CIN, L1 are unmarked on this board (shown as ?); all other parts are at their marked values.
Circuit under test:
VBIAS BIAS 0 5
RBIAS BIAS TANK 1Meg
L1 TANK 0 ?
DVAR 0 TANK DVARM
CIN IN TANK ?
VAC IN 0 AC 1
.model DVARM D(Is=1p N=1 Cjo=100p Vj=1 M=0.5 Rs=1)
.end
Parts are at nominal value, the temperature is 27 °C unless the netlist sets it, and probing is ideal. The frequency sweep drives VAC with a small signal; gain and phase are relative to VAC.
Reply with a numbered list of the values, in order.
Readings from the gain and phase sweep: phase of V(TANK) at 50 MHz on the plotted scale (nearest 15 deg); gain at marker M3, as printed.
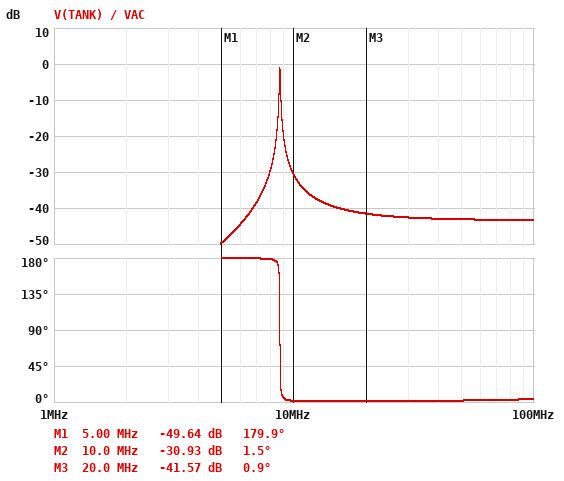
1. 0 deg
2. -41.57 dB
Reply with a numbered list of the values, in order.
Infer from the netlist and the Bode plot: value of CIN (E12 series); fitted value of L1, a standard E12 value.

1. 680 fF
2. 3.3 µH
